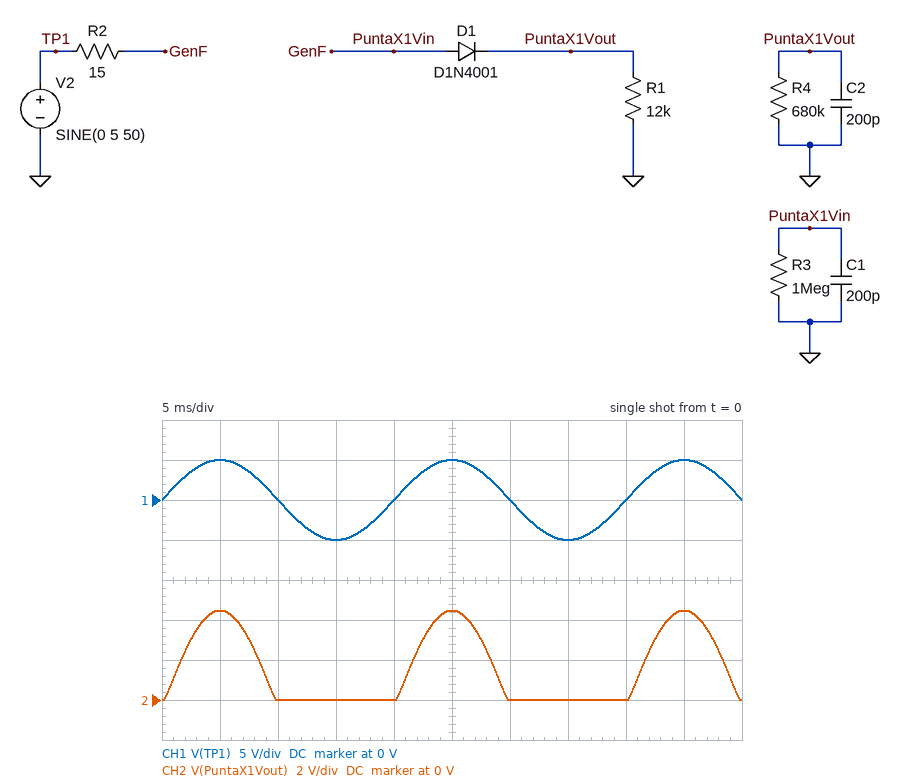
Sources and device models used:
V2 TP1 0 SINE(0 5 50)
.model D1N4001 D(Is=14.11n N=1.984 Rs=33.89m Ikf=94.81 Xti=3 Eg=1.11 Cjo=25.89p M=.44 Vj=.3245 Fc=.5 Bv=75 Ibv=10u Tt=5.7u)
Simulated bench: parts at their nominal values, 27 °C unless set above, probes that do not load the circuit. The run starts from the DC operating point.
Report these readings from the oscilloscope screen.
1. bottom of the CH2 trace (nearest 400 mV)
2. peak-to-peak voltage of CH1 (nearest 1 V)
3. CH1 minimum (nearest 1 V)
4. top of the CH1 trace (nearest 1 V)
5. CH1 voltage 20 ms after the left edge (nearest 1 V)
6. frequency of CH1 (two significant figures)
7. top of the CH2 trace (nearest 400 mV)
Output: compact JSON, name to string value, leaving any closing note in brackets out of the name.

{"bottom of the CH2 trace": "0 V", "peak-to-peak voltage of CH1": "10 V", "CH1 minimum": "-5 V", "top of the CH1 trace": "5 V", "CH1 voltage 20 ms after the left edge": "0 V", "frequency of CH1": "50 Hz", "top of the CH2 trace": "4.4 V"}
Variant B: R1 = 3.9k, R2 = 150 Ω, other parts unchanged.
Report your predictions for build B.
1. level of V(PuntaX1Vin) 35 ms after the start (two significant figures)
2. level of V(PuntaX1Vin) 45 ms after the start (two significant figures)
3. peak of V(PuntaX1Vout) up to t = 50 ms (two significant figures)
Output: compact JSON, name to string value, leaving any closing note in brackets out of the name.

{"level of V(PuntaX1Vin) 35 ms after the start": "-5.0 V", "level of V(PuntaX1Vin) 45 ms after the start": "4.8 V", "peak of V(PuntaX1Vout) up to t = 50 ms": "4.3 V"}
